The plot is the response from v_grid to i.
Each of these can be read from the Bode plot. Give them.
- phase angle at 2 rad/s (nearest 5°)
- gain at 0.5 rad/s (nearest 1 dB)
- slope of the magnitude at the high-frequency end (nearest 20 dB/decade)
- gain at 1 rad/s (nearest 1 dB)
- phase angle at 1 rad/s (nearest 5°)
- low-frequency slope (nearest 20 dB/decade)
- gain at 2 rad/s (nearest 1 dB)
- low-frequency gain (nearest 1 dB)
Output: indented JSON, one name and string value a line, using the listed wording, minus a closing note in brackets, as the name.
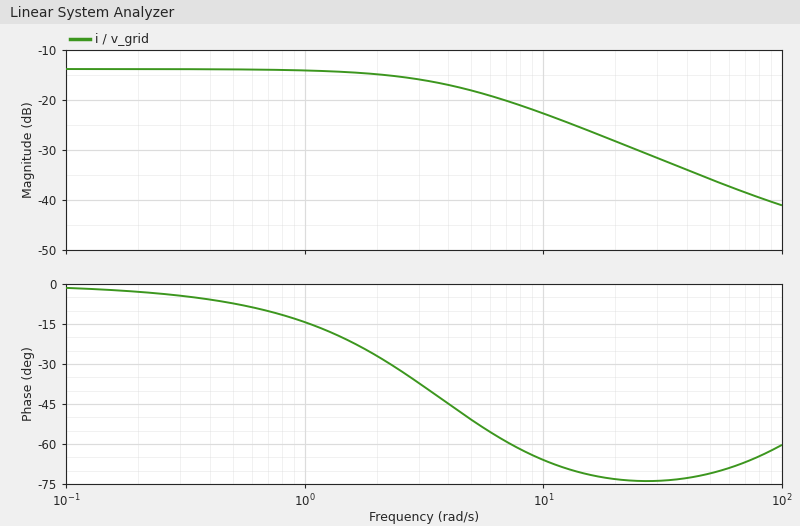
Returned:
{
  "phase angle at 2 rad/s": "-25°",
  "gain at 0.5 rad/s": "-14 dB",
  "slope of the magnitude at the high-frequency end": "-20 dB/decade",
  "gain at 1 rad/s": "-14 dB",
  "phase angle at 1 rad/s": "-15°",
  "low-frequency slope": "0 dB/decade",
  "gain at 2 rad/s": "-15 dB",
  "low-frequency gain": "-14 dB"
}
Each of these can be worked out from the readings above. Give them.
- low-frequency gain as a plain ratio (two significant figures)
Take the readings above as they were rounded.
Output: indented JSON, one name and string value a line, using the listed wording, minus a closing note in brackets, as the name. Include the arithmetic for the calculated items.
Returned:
{
  "low-frequency gain as a plain ratio": "10^(-14 / 20) = 0.20"
}
